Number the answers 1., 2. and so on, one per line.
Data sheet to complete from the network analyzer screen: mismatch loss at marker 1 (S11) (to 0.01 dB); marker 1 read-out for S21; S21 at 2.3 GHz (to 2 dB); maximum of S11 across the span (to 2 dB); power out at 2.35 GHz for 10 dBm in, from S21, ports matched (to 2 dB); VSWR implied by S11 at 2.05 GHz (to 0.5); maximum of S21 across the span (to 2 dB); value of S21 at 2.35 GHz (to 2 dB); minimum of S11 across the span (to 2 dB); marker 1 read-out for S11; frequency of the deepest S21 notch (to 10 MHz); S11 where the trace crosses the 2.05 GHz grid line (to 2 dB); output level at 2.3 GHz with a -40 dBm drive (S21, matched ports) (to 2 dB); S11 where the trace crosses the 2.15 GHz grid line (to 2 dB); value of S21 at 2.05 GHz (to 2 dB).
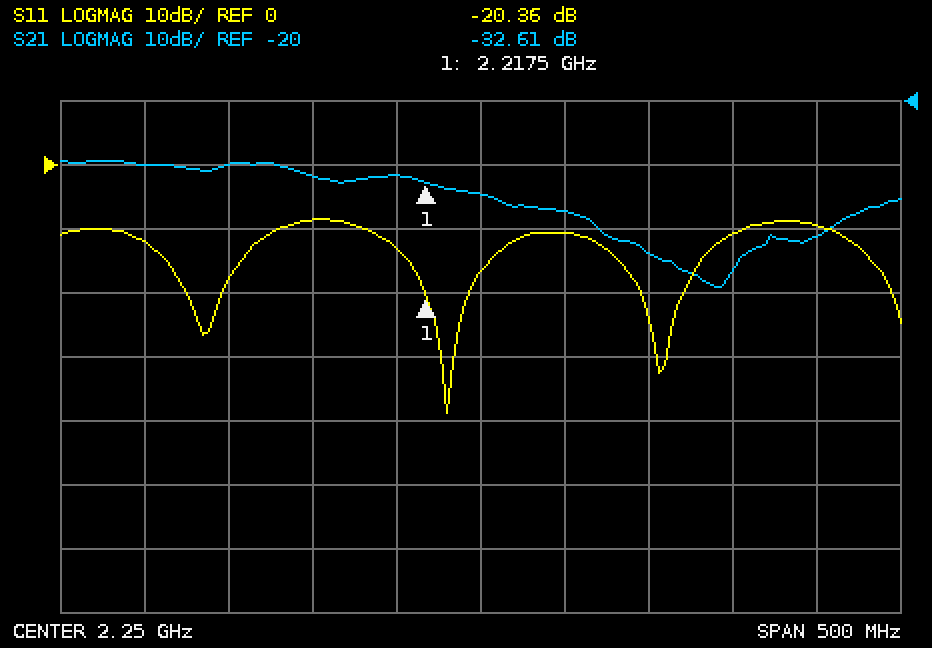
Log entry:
1. 0.04 dB
2. -32.61 dB
3. -38 dB
4. -8 dB
5. -34 dBm
6. 1.5
7. -30 dB
8. -44 dB
9. -38 dB
10. -20.36 dB
11. 2.39 GHz
12. -12 dB
13. -78 dBm
14. -8 dB
15. -30 dB
